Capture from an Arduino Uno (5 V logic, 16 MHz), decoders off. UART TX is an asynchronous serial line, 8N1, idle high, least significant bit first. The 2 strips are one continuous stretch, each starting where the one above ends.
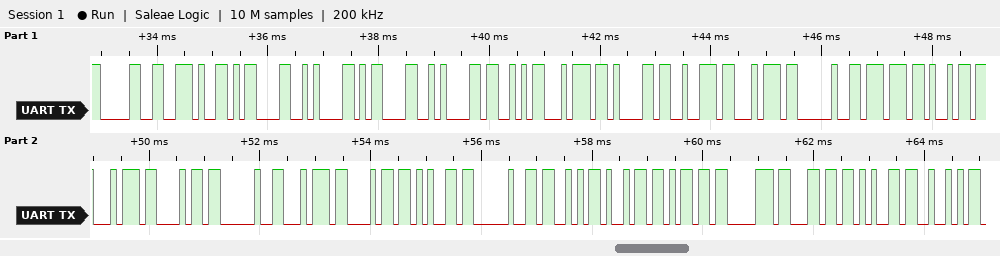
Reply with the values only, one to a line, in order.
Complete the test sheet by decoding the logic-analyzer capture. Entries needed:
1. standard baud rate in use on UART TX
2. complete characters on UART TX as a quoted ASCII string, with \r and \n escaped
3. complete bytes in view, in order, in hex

9600 baud
"0.\r\n\r\nStart with the SimpleR"
30 2E 0D 0A 0D 0A 53 74 61 72 74 20 77 69 74 68 20 74 68 65 20 53 69 6D 70 6C 65 52
